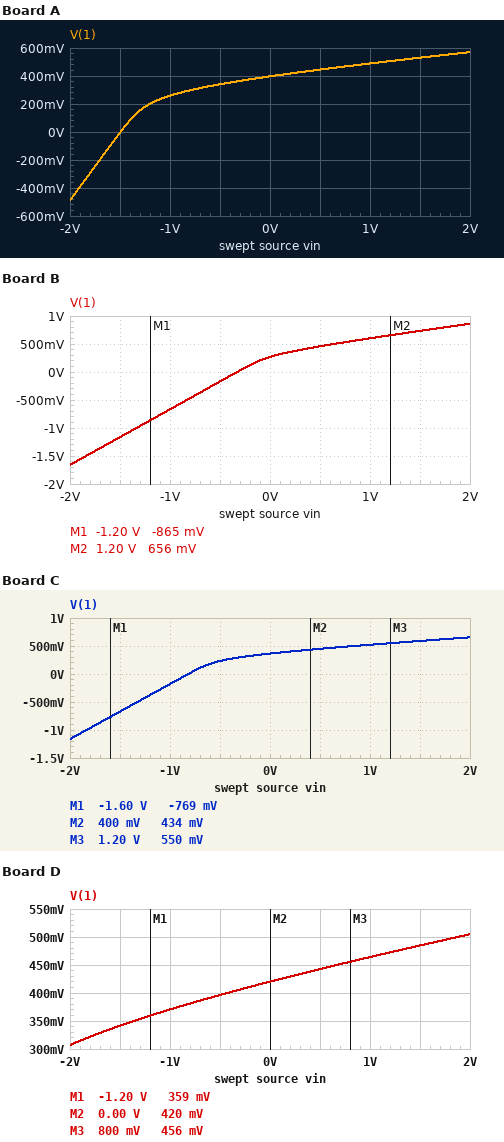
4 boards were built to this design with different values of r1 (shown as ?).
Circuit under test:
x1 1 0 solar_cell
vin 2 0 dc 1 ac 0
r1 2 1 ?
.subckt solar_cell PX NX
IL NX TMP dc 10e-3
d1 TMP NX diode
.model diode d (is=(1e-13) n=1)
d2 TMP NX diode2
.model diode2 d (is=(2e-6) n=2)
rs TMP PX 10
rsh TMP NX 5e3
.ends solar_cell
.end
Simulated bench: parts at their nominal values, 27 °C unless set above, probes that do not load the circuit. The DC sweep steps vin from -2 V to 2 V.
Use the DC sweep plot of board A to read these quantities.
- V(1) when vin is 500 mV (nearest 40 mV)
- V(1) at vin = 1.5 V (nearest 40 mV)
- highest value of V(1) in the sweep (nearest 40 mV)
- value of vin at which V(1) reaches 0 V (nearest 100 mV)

440 mV
520 mV
560 mV
-1.5 V
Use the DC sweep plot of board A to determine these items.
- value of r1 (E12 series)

150 Ω
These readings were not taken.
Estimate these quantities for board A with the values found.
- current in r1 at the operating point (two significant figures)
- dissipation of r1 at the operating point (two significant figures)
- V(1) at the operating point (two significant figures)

3.4 mA
1.7 mW
490 mV
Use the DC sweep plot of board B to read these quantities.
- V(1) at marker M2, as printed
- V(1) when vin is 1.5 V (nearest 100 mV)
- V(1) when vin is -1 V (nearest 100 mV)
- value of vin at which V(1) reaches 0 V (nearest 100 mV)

656 mV
700 mV
-700 mV
-300 mV
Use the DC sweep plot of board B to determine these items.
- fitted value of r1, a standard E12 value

33 Ω
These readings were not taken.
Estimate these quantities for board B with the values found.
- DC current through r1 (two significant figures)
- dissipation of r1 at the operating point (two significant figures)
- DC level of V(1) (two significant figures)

12 mA
4.8 mW
600 mV
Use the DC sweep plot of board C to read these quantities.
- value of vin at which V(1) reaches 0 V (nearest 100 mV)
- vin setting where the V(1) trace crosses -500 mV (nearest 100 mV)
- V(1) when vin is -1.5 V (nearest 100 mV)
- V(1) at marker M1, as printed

-800 mV
-1.3 V
-700 mV
-769 mV
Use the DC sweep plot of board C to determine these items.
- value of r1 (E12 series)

82 Ω
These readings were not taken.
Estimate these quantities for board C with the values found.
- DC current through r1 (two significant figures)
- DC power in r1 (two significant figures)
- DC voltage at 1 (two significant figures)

5.8 mA
2.8 mW
520 mV
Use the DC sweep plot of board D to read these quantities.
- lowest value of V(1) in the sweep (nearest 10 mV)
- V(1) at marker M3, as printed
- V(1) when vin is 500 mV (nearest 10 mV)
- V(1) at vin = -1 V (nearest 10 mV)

310 mV
456 mV
440 mV
370 mV
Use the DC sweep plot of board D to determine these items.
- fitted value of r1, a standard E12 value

330 Ω
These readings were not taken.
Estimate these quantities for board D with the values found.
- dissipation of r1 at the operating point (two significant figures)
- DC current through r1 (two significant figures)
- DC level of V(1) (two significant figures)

870 µW
1.6 mA
460 mV
